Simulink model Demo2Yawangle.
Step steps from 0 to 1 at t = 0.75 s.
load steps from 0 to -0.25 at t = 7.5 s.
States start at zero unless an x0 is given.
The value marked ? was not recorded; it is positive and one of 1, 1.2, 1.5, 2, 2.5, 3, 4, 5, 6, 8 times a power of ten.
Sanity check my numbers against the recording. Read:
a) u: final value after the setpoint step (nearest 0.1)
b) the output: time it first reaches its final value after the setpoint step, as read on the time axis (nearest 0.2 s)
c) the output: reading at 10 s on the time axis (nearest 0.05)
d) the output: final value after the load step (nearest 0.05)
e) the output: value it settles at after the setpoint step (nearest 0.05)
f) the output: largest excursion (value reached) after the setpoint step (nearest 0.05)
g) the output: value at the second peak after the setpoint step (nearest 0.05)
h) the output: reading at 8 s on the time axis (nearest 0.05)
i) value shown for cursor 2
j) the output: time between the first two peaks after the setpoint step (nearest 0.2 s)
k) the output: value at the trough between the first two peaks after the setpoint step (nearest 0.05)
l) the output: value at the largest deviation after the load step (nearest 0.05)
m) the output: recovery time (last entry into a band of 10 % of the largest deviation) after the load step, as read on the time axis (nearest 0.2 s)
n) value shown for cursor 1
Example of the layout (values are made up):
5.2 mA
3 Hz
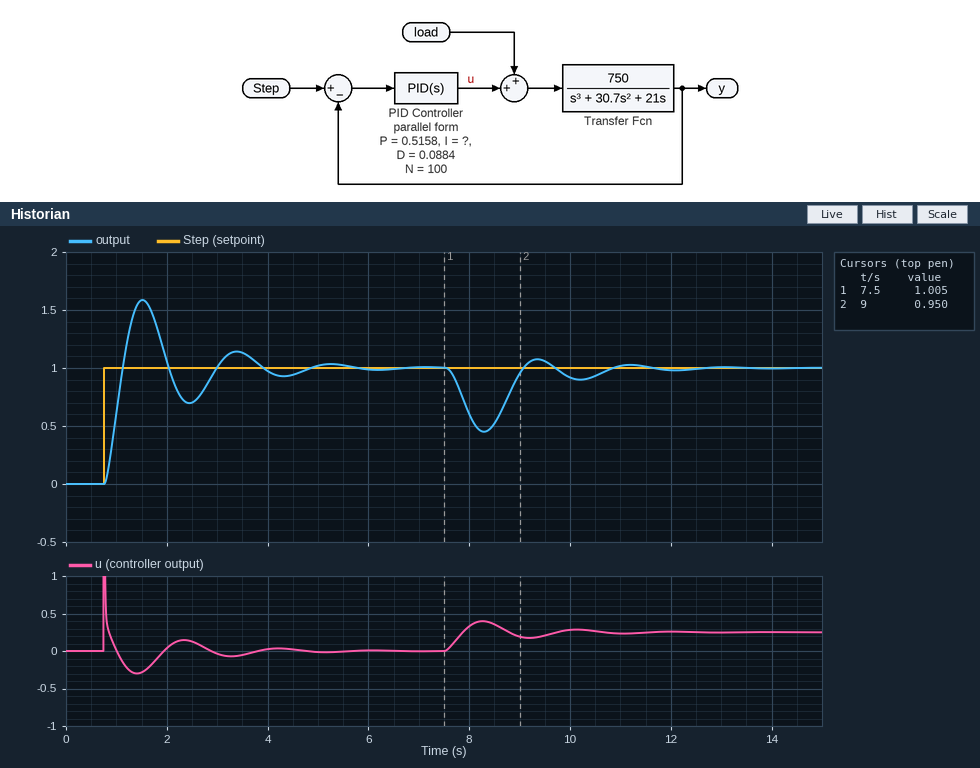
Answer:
0.0
1.2 s
0.90
1.00
1.00
1.60
1.15
0.60
0.950
1.8 s
0.70
0.45
10.6 s
1.005
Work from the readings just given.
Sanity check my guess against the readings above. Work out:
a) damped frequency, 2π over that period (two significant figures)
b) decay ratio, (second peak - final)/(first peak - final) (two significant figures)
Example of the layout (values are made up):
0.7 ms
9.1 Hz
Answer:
3.5 rad/s
0.25
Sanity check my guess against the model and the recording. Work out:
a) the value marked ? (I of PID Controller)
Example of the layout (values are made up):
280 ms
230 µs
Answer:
0.5
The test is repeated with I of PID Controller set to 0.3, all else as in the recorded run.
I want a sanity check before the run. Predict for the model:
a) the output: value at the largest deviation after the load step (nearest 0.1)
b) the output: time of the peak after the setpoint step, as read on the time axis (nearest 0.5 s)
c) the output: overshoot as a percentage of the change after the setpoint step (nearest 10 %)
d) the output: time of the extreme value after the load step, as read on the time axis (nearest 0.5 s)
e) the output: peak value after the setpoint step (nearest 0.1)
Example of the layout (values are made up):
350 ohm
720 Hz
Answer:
0.4
1.5 s
50 %
8.5 s
1.5
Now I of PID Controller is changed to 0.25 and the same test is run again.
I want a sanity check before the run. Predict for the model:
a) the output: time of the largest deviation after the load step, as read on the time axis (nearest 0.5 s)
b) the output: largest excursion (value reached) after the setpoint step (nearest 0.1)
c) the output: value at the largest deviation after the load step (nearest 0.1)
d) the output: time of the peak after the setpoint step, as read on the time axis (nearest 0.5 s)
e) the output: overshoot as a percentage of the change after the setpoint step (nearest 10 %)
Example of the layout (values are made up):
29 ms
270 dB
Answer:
8.5 s
1.5
0.4
1.5 s
50 %
